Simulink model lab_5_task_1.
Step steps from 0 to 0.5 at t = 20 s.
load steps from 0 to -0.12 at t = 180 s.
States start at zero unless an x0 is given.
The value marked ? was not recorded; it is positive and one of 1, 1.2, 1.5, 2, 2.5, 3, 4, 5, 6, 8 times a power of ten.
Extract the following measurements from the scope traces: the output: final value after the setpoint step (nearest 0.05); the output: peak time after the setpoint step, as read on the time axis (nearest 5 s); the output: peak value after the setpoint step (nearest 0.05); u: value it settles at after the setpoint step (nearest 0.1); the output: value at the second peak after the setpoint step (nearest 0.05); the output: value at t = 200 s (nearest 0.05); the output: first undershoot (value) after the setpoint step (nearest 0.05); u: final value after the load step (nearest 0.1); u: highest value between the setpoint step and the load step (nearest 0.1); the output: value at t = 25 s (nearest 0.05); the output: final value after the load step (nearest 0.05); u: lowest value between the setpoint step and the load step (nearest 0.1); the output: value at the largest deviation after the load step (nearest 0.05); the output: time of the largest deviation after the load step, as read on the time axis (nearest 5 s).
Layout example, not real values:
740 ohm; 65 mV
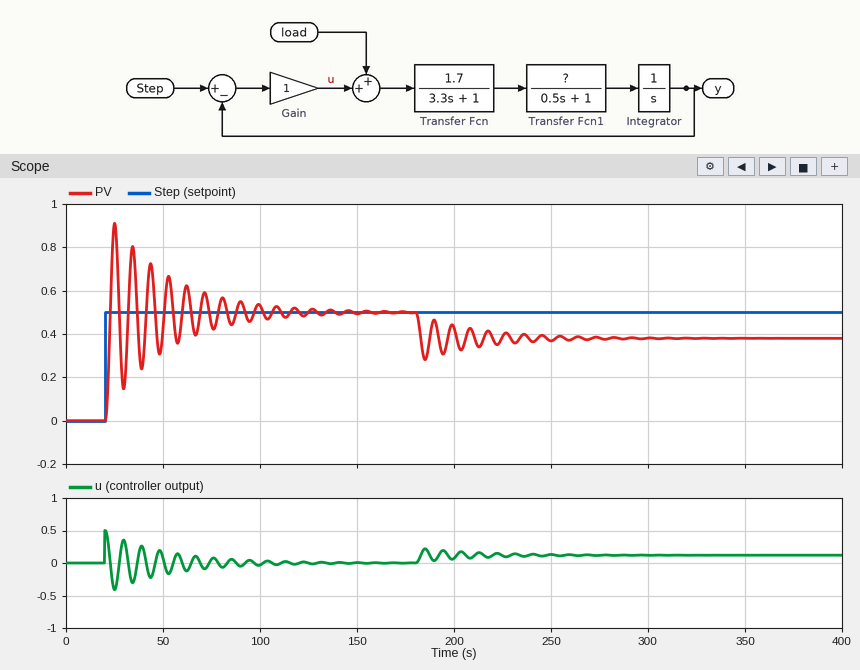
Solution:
0.50; 25 s; 0.90; 0.0; 0.80; 0.45; 0.15; 0.1; 0.5; 0.90; 0.40; -0.4; 0.30; 185 s
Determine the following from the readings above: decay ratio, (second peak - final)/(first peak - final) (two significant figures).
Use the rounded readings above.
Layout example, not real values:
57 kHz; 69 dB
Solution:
0.75
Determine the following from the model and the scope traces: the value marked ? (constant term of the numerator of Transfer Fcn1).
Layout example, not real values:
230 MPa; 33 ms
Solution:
1
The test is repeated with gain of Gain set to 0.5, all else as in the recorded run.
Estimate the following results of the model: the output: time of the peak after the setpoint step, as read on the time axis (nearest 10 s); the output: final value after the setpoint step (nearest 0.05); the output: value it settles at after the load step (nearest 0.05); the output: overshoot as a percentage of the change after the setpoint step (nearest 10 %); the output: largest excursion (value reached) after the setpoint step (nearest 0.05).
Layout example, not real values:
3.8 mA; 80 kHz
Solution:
30 s; 0.50; 0.25; 60 %; 0.80
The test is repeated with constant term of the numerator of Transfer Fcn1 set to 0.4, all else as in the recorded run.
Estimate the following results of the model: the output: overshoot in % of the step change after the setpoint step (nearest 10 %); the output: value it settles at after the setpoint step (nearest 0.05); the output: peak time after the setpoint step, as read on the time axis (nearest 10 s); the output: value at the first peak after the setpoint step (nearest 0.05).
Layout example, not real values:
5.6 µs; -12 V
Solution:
50 %; 0.50; 30 s; 0.75
